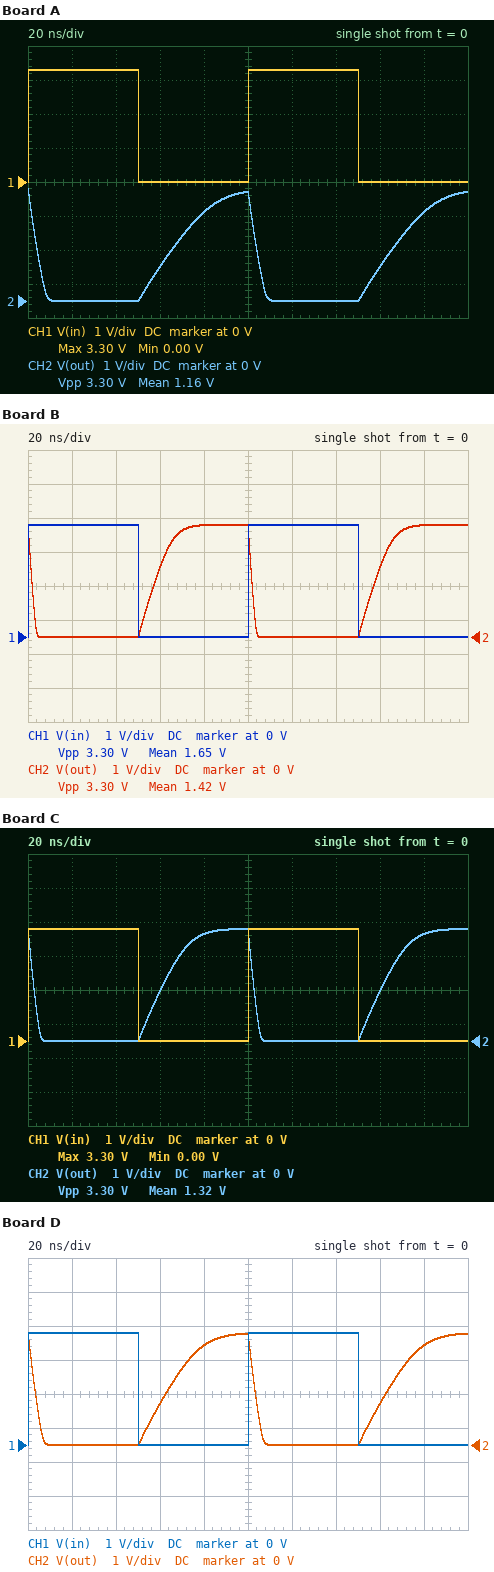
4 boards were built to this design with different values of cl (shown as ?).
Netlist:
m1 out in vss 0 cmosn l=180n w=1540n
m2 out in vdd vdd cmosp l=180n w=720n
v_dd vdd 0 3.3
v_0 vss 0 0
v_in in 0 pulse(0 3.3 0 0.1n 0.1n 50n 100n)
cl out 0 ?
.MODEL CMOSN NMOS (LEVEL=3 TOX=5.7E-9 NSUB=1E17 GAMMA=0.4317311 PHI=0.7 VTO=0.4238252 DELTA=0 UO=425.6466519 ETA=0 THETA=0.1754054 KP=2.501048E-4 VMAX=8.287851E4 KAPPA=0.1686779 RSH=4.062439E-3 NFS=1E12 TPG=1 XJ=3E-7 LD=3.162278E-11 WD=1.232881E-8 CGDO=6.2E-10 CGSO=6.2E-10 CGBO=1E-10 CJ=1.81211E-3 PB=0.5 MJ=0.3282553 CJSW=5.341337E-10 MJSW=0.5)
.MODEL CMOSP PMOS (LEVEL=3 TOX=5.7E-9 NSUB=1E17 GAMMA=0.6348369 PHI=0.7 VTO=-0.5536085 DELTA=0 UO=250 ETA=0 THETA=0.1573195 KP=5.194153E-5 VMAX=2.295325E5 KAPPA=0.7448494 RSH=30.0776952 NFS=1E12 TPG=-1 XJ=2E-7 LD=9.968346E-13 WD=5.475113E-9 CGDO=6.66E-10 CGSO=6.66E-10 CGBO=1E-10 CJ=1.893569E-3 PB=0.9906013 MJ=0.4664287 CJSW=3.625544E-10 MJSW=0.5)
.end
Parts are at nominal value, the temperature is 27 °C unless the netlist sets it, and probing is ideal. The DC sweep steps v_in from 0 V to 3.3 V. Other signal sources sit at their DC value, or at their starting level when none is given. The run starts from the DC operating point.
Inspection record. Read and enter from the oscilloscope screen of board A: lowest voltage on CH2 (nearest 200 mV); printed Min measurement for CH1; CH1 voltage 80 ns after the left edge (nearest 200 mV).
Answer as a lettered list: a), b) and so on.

a) 0 V
b) 0.00 V
c) 0 V
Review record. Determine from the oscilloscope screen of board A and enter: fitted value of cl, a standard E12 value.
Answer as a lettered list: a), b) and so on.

a) 3.3 pF
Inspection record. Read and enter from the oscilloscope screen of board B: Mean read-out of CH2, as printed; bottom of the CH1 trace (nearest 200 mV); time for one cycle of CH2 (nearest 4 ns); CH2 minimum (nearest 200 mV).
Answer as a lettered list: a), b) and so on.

a) 1.42 V
b) 0 V
c) 100 ns
d) 0 V
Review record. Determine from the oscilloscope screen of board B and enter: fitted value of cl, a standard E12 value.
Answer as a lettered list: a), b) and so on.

a) 1.5 pF
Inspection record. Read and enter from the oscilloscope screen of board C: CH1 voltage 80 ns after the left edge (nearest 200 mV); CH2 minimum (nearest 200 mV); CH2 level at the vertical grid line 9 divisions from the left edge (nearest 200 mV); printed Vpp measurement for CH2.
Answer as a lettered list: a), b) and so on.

a) 0 V
b) 0 V
c) 3.2 V
d) 3.30 V
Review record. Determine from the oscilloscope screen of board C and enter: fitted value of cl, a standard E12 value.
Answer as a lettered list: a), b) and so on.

a) 2.2 pF
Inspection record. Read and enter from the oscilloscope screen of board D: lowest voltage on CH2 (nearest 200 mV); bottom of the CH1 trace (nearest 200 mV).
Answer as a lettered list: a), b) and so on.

a) 0 V
b) 0 V
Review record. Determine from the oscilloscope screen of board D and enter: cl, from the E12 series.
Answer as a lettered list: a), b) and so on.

a) 2.7 pF
